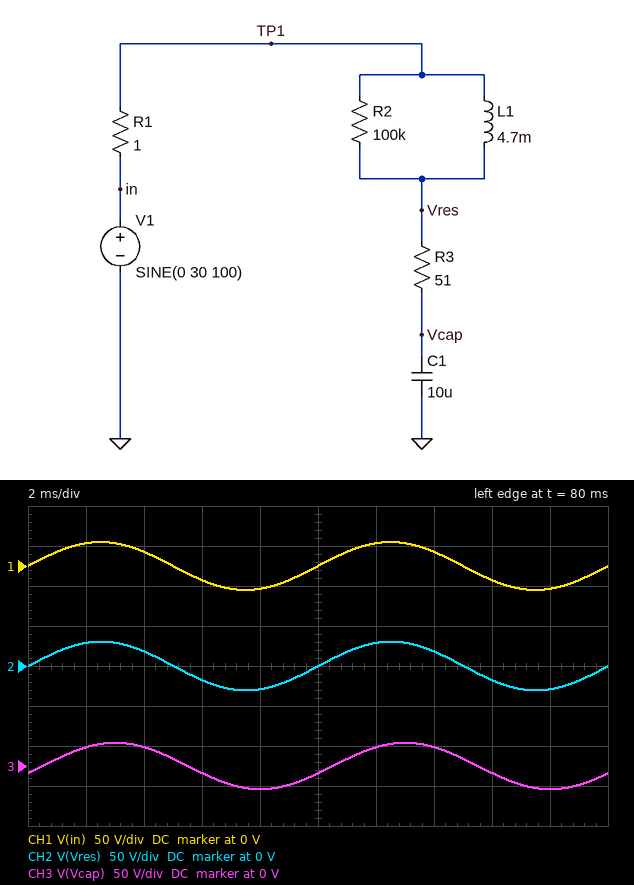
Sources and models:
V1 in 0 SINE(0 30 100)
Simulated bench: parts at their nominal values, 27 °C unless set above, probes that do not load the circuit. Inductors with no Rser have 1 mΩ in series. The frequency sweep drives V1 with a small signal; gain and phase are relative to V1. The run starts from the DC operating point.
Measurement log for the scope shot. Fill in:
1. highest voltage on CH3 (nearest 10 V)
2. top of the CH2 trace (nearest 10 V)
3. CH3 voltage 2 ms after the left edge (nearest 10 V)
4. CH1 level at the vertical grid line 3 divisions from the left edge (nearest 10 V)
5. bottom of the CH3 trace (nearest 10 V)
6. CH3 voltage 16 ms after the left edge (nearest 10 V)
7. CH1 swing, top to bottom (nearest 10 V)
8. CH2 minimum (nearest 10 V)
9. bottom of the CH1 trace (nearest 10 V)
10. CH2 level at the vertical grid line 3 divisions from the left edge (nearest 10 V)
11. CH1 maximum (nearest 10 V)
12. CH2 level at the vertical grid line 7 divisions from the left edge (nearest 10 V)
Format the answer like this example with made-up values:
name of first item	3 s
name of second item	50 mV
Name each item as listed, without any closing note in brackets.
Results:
highest voltage on CH3	30 V
top of the CH2 trace	30 V
CH3 voltage 2 ms after the left edge	20 V
CH1 level at the vertical grid line 3 divisions from the left edge	-20 V
bottom of the CH3 trace	-30 V
CH3 voltage 16 ms after the left edge	-10 V
CH1 swing, top to bottom	60 V
CH2 minimum	-30 V
bottom of the CH1 trace	-30 V
CH2 level at the vertical grid line 3 divisions from the left edge	-20 V
CH1 maximum	30 V
CH2 level at the vertical grid line 7 divisions from the left edge	20 V
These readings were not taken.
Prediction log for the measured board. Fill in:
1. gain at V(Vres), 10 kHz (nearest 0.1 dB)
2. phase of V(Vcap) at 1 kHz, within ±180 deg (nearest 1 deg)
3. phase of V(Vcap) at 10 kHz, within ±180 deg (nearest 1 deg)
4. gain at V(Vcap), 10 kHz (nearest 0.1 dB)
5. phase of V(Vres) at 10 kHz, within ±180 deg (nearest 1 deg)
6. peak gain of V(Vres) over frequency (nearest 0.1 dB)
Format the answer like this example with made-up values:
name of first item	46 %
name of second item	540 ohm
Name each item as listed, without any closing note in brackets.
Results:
gain at V(Vres), 10 kHz	-15.3 dB
phase of V(Vcap) at 1 kHz, within ±180 deg	-105 deg
phase of V(Vcap) at 10 kHz, within ±180 deg	-170 deg
gain at V(Vcap), 10 kHz	-45.5 dB
phase of V(Vres) at 10 kHz, within ±180 deg	-82 deg
peak gain of V(Vres) over frequency	0.8 dB
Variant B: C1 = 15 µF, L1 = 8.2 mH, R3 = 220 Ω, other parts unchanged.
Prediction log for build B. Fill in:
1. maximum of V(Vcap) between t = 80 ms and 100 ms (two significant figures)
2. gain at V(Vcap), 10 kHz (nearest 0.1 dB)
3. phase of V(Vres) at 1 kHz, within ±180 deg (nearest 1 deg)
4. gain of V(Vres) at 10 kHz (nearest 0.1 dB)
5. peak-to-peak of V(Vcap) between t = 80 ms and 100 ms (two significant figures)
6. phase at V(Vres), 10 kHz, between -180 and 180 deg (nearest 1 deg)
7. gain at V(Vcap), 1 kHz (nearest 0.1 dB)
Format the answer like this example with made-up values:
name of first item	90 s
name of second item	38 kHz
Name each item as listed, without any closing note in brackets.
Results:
maximum of V(Vcap) between t = 80 ms and 100 ms	13 V
gain at V(Vcap), 10 kHz	-54.5 dB
phase of V(Vres) at 1 kHz, within ±180 deg	-13 deg
gain of V(Vres) at 10 kHz	-8.1 dB
peak-to-peak of V(Vcap) between t = 80 ms and 100 ms	26 V
phase at V(Vres), 10 kHz, between -180 and 180 deg	-67 deg
gain at V(Vcap), 1 kHz	-26.5 dB
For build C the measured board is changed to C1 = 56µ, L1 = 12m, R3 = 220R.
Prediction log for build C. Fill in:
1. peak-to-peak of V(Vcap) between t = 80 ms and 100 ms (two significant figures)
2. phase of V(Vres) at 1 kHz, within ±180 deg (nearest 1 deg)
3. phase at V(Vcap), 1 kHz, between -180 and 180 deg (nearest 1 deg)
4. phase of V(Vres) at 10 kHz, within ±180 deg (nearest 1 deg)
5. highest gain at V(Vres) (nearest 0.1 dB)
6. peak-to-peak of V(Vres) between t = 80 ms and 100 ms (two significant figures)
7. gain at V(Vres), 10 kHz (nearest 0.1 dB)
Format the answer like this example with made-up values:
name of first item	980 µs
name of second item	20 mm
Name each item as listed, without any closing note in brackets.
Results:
peak-to-peak of V(Vcap) between t = 80 ms and 100 ms	7.7 V
phase of V(Vres) at 1 kHz, within ±180 deg	-19 deg
phase at V(Vcap), 1 kHz, between -180 and 180 deg	-108 deg
phase of V(Vres) at 10 kHz, within ±180 deg	-73 deg
highest gain at V(Vres)	0 dB
peak-to-peak of V(Vres) between t = 80 ms and 100 ms	60 V
gain at V(Vres), 10 kHz	-11.1 dB
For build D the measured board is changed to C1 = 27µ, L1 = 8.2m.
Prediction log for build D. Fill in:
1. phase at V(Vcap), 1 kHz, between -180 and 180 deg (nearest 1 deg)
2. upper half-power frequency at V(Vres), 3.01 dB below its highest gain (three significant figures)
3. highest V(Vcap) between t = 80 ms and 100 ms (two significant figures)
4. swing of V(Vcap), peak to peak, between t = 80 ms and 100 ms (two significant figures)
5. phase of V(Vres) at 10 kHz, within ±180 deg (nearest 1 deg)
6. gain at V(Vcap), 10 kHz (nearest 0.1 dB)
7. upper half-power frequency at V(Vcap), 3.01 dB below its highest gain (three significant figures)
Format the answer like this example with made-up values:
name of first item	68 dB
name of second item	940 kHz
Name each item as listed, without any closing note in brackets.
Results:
phase at V(Vcap), 1 kHz, between -180 and 180 deg	-131 deg
upper half-power frequency at V(Vres), 3.01 dB below its highest gain	977 Hz
highest V(Vcap) between t = 80 ms and 100 ms	24 V
swing of V(Vcap), peak to peak, between t = 80 ms and 100 ms	47 V
phase of V(Vres) at 10 kHz, within ±180 deg	-85 deg
gain at V(Vcap), 10 kHz	-58.9 dB
upper half-power frequency at V(Vcap), 3.01 dB below its highest gain	127 Hz
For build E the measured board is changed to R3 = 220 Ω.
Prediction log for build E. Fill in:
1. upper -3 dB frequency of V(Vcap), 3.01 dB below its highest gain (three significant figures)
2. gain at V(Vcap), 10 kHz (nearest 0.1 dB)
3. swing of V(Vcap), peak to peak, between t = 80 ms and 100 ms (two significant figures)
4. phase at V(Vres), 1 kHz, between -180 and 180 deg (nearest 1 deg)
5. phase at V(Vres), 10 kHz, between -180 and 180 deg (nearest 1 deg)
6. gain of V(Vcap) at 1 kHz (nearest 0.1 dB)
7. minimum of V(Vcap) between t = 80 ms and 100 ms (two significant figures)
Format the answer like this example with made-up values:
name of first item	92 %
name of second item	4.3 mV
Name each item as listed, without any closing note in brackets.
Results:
upper -3 dB frequency of V(Vcap), 3.01 dB below its highest gain	72.7 Hz
gain at V(Vcap), 10 kHz	-47.3 dB
swing of V(Vcap), peak to peak, between t = 80 ms and 100 ms	35 V
phase at V(Vres), 1 kHz, between -180 and 180 deg	-8 deg
phase at V(Vres), 10 kHz, between -180 and 180 deg	-53 deg
gain of V(Vcap) at 1 kHz	-22.9 dB
minimum of V(Vcap) between t = 80 ms and 100 ms	-18 V
